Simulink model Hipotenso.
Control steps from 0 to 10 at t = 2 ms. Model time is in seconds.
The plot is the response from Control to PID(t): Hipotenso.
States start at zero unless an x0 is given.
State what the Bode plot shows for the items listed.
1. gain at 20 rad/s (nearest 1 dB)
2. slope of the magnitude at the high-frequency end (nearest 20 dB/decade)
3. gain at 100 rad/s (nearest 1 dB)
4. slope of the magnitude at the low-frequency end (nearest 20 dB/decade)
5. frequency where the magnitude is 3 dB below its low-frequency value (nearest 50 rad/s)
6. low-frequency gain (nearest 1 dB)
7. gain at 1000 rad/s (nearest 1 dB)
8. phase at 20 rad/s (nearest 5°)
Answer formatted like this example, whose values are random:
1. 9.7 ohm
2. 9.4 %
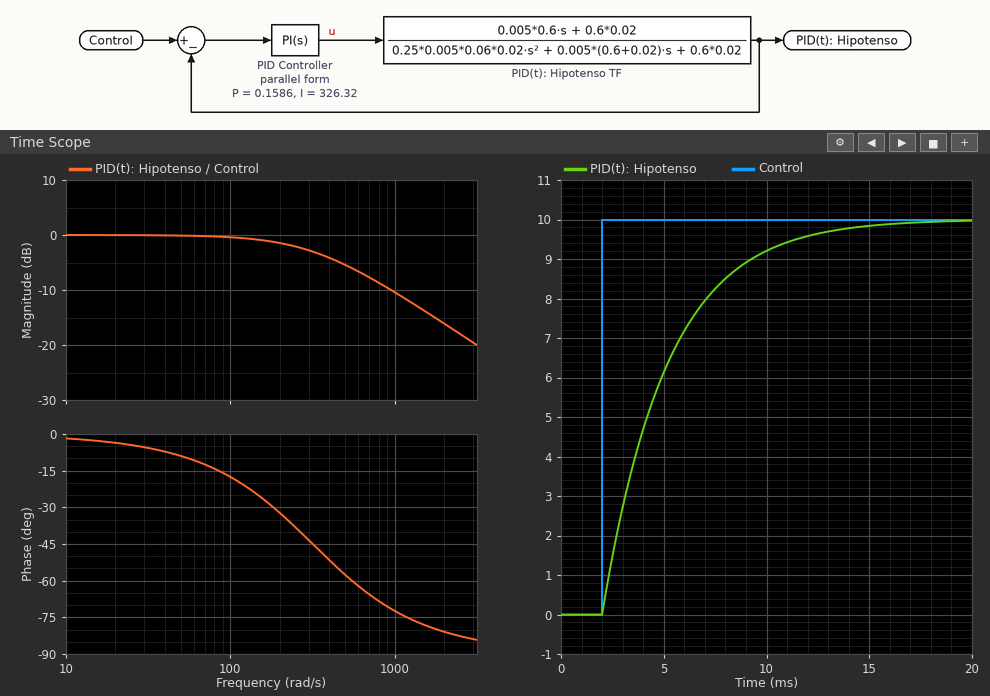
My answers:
1. 0 dB
2. -20 dB/decade
3. 0 dB
4. 0 dB/decade
5. 300 rad/s
6. 0 dB
7. -10 dB
8. -5°
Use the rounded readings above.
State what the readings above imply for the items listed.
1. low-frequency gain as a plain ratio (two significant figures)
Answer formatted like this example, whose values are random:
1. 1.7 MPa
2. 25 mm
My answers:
1. 1.0
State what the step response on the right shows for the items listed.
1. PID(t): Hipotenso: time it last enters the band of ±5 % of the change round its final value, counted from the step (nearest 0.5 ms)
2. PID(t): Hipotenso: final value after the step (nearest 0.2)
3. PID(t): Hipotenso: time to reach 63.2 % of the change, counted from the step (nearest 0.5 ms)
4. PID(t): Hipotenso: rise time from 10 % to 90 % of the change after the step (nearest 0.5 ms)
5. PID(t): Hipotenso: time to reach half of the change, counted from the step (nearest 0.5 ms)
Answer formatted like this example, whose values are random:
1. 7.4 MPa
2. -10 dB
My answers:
1. 9.5 ms
2. 10.0
3. 3.0 ms
4. 7.0 ms
5. 2.0 ms
